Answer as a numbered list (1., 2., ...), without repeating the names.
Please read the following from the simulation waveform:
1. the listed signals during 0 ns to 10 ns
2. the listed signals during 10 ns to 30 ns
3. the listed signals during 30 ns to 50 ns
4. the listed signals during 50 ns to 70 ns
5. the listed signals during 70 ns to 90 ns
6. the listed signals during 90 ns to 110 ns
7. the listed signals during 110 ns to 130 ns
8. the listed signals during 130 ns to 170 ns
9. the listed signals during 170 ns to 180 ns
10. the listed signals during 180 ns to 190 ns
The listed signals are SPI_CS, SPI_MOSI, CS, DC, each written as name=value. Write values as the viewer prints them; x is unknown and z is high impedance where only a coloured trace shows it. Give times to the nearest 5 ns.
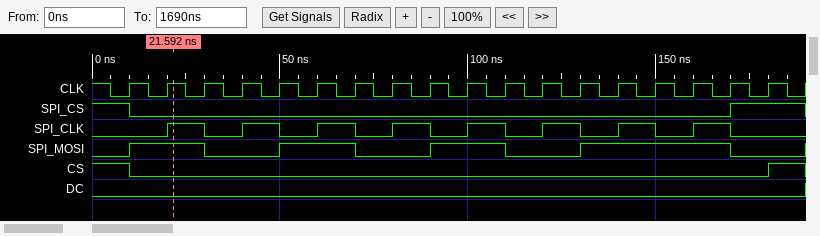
1. SPI_CS=1, SPI_MOSI=0, CS=1, DC=0
2. SPI_CS=0, SPI_MOSI=1, CS=0, DC=0
3. SPI_CS=0, SPI_MOSI=0, CS=0, DC=0
4. SPI_CS=0, SPI_MOSI=1, CS=0, DC=0
5. SPI_CS=0, SPI_MOSI=0, CS=0, DC=0
6. SPI_CS=0, SPI_MOSI=1, CS=0, DC=0
7. SPI_CS=0, SPI_MOSI=0, CS=0, DC=0
8. SPI_CS=0, SPI_MOSI=1, CS=0, DC=0
9. SPI_CS=1, SPI_MOSI=0, CS=0, DC=0
10. SPI_CS=1, SPI_MOSI=0, CS=1, DC=0
